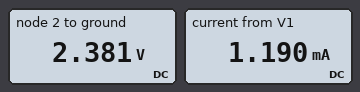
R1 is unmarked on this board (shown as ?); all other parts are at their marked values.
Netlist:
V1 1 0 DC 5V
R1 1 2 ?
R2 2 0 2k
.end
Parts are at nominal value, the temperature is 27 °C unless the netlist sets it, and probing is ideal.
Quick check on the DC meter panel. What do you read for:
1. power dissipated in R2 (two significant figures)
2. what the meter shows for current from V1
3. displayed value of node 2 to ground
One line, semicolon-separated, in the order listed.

2.8 mW; 1.190 mA; 2.381 V
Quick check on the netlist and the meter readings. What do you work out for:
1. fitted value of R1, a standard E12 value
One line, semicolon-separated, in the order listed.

2.2 kΩ
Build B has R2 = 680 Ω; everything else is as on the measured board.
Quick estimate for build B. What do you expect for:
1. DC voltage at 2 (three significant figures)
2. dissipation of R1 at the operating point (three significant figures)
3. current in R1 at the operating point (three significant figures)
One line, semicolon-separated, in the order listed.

1.18 V; 6.63 mW; 1.74 mA
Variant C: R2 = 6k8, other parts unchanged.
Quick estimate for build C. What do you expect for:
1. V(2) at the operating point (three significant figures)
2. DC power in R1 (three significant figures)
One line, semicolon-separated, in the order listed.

3.78 V; 679 µW
